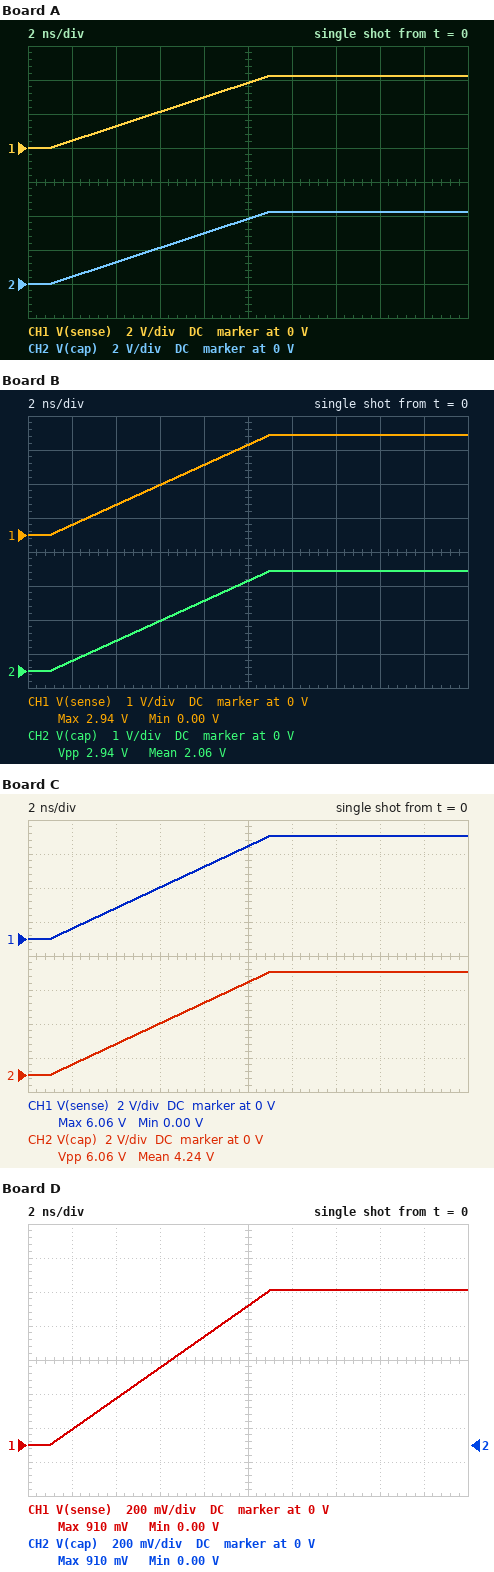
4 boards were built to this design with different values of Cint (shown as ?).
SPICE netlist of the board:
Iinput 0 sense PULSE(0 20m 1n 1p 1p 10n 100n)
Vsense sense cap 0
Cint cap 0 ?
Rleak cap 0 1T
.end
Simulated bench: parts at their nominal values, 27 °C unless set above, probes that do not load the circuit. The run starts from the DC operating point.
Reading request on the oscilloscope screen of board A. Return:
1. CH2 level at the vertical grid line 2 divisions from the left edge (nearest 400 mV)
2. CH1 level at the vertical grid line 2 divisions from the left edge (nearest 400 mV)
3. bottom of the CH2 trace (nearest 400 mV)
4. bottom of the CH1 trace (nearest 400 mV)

1.2 V
1.2 V
0 V
0 V
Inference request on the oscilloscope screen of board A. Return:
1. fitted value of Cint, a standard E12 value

47 pF
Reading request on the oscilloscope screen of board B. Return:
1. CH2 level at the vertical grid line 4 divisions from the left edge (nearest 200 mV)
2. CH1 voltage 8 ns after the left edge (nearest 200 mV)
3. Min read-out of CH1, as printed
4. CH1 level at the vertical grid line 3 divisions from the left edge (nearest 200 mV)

2.0 V
2.0 V
0.00 V
1.4 V
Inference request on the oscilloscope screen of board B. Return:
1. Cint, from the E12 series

68 pF
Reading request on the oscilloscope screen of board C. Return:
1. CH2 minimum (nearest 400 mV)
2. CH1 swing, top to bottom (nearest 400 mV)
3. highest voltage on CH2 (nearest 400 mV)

0 V
6.0 V
6.0 V
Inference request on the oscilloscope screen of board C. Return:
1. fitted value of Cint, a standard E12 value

33 pF
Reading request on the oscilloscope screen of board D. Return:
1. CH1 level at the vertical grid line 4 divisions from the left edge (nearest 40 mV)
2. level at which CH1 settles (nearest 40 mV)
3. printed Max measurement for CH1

640 mV
920 mV
910 mV
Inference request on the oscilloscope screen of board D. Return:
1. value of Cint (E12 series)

220 pF
